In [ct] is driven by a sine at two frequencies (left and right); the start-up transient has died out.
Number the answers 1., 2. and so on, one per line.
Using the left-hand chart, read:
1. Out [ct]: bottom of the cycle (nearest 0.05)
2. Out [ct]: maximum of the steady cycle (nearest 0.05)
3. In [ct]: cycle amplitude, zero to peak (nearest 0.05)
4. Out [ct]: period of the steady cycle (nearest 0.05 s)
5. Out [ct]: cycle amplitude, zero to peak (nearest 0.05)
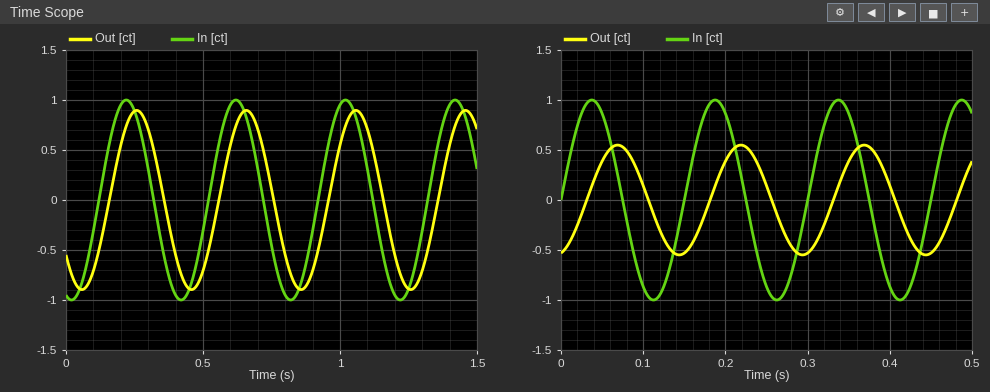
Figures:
1. -0.90
2. 0.90
3. 1.00
4. 0.40 s
5. 0.90
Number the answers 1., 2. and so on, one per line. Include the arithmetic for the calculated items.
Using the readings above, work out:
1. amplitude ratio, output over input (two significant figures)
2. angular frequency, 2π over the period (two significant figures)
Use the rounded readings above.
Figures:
1. 0.9 / 1 = 0.90
2. 2π / 0.4 = 16 rad/s
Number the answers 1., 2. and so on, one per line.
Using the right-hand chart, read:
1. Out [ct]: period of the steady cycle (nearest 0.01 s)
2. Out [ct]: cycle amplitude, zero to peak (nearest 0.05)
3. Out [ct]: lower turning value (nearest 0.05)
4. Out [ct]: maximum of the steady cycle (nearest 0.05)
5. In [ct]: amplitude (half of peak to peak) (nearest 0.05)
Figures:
1. 0.15 s
2. 0.55
3. -0.55
4. 0.55
5. 1.00
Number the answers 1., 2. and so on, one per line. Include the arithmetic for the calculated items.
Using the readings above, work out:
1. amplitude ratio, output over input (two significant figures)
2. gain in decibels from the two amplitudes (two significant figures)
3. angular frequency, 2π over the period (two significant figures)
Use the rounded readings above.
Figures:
1. 0.55 / 1 = 0.55
2. 20 log10(0.55 / 1) = -5.2 dB
3. 2π / 0.15 = 42 rad/s
